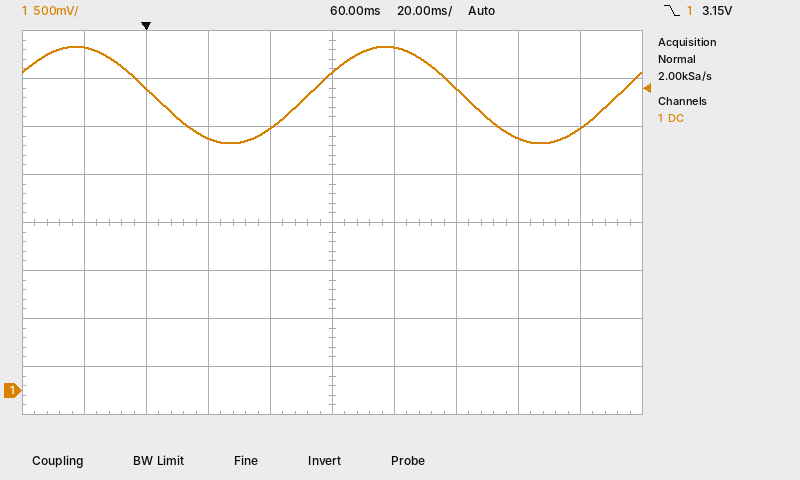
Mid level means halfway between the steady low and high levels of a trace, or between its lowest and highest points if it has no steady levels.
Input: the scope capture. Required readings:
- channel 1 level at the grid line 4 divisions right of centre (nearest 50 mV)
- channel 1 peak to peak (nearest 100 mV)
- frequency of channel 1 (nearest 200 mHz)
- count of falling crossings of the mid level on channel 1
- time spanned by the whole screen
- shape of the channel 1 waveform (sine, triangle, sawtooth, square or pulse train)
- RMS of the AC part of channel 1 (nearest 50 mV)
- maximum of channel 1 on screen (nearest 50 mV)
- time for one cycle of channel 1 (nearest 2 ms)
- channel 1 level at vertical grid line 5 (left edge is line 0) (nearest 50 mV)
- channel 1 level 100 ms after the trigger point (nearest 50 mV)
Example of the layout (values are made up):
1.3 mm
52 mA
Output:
2.75 V
1.00 V
10.0 Hz
2
200 ms
sine
350 mV
3.60 V
100 ms
3.30 V
3.15 V
